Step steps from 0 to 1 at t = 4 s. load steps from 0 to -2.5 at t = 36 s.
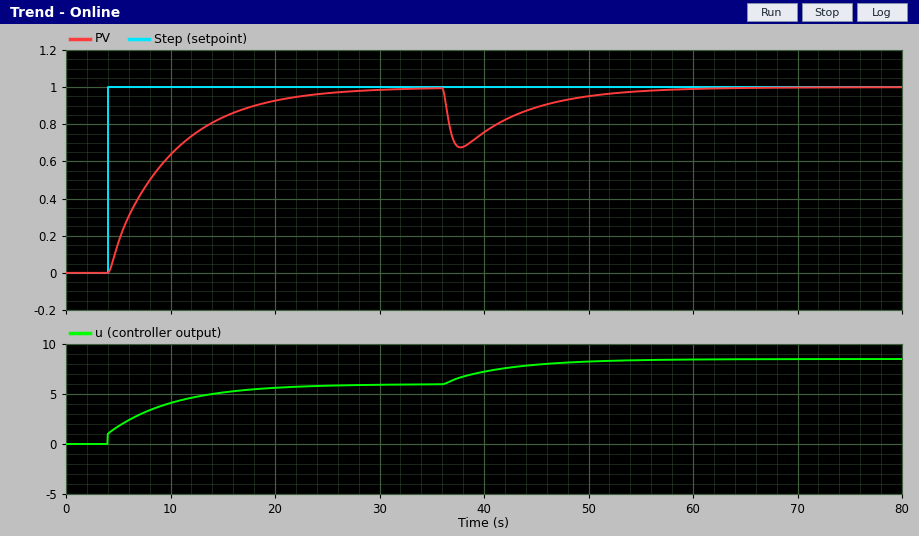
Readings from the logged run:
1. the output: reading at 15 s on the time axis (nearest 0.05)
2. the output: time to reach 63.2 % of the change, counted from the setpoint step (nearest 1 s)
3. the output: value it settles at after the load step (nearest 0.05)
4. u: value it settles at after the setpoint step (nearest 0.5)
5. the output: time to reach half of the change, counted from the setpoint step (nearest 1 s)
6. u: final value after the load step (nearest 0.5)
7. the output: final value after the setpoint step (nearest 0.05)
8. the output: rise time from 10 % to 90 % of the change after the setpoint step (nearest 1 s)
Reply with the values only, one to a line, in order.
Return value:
0.85
6 s
1.00
6.0
4 s
8.5
1.00
13 s
